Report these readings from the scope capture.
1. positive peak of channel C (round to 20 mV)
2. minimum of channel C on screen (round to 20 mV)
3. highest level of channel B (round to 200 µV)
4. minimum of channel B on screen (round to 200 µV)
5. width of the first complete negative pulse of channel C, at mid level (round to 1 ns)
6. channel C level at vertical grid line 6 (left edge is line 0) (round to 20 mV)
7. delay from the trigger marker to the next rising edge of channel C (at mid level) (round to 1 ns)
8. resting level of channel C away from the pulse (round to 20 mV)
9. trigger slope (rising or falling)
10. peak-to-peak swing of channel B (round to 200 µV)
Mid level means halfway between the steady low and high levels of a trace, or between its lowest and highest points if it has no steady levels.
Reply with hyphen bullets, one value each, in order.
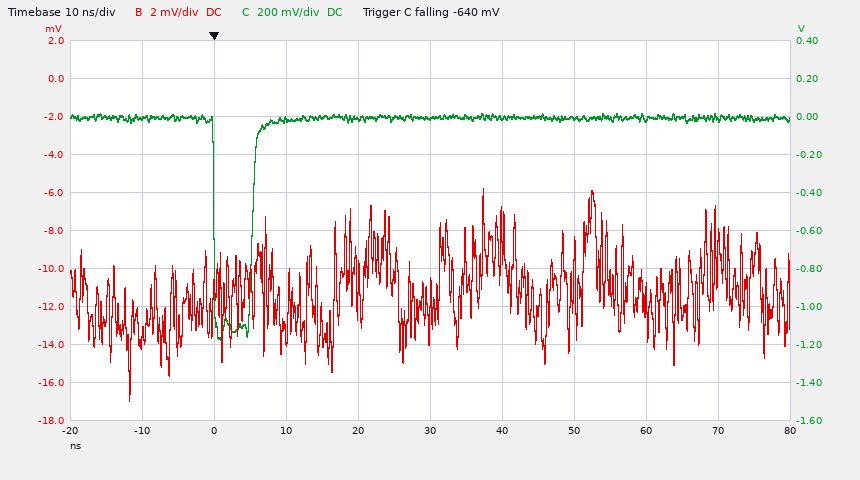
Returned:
- 20 mV
- -1.18 V
- -5.8 mV
- -17.0 mV
- 5 ns
- 0 mV
- 5 ns
- 0 mV
- falling
- 11.2 mV
